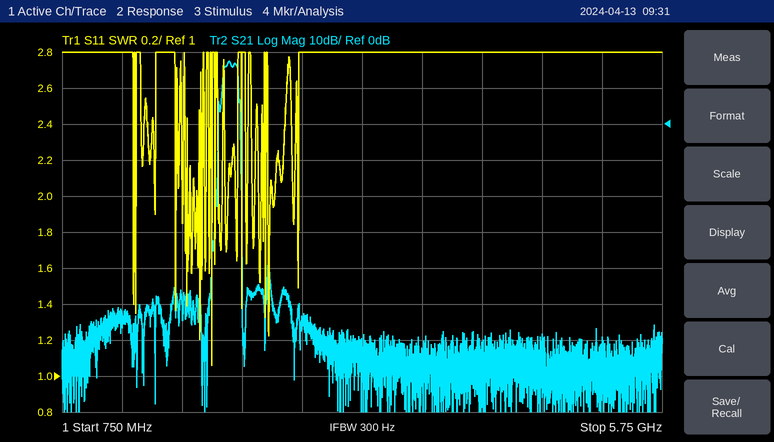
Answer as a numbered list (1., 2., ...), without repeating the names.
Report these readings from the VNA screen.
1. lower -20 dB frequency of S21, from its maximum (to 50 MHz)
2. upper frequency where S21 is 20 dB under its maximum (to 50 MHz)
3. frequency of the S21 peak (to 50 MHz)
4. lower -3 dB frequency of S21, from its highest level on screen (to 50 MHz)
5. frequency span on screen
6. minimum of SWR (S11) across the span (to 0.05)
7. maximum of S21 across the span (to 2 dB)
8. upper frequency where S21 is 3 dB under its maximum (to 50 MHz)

1. 2.05 GHz
2. 2.25 GHz
3. 2.15 GHz
4. 2.10 GHz
5. 5 GHz
6. 1.05
7. 18 dB
8. 2.20 GHz
